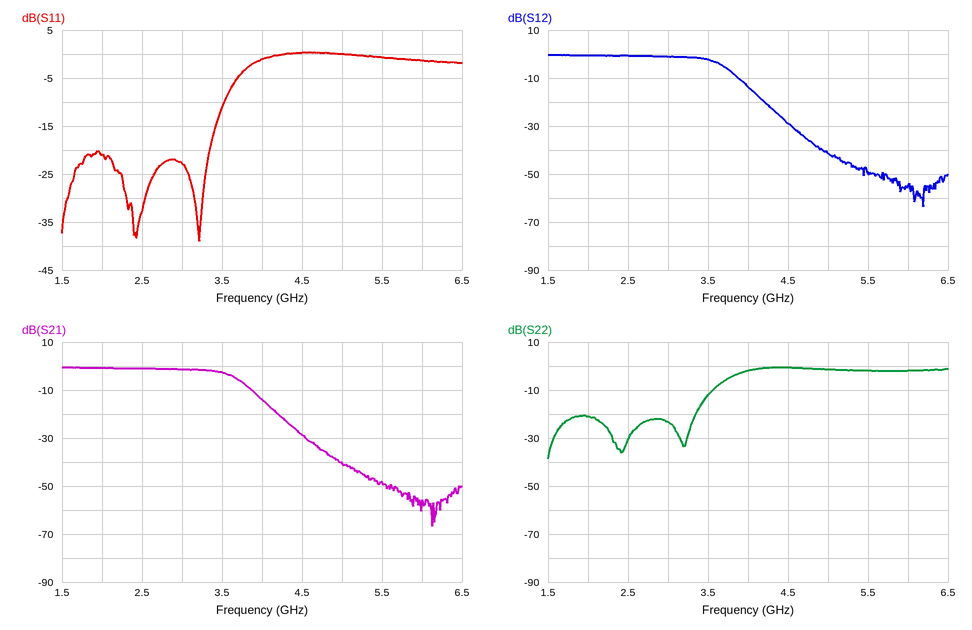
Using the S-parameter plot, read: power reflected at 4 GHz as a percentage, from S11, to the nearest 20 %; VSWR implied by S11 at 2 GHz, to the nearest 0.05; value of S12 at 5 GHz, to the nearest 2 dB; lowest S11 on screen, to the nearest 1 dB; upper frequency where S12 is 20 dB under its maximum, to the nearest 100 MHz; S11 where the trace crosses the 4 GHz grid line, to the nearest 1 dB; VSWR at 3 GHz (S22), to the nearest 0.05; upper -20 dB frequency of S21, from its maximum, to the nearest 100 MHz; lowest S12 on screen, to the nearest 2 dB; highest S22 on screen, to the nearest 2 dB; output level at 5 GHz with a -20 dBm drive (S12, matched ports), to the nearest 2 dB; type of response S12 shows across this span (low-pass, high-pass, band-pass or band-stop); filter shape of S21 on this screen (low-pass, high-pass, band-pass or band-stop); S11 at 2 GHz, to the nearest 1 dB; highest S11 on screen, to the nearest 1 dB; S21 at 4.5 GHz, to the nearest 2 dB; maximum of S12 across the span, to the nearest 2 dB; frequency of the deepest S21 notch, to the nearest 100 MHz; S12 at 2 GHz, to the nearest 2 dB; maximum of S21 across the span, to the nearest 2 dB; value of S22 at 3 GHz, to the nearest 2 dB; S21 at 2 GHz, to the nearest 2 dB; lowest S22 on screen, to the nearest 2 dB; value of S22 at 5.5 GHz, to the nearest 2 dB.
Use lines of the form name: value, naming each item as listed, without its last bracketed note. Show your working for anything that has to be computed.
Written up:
power reflected at 4 GHz as a percentage, from S11, to the nearest 20 %: 10^(-1/10) ≈ 79.4 %, so 80 % to the nearest 20 %
VSWR implied by S11 at 2 GHz, to the nearest 0.05: |Γ| = 10^(-21/20) = 0.0891; VSWR = (1 + 0.0891)/(1 − 0.0891) ≈ 1.20
value of S12 at 5 GHz, to the nearest 2 dB: -42 dB
lowest S11 on screen, to the nearest 1 dB: -39 dB
upper frequency where S12 is 20 dB under its maximum, to the nearest 100 MHz: 4.2 GHz
S11 where the trace crosses the 4 GHz grid line, to the nearest 1 dB: -1 dB
VSWR at 3 GHz (S22), to the nearest 0.05: |Γ| = 10^(-24/20) = 0.0631; VSWR = (1 + 0.0631)/(1 − 0.0631) ≈ 1.13, so 1.15 to the nearest 0.05
upper -20 dB frequency of S21, from its maximum, to the nearest 100 MHz: 4.2 GHz
lowest S12 on screen, to the nearest 2 dB: -64 dB
highest S22 on screen, to the nearest 2 dB: 0 dB
output level at 5 GHz with a -20 dBm drive (S12, matched ports), to the nearest 2 dB: -20 dBm + (-42 dB) = -62 dBm
type of response S12 shows across this span: low-pass
filter shape of S21 on this screen: low-pass
S11 at 2 GHz, to the nearest 1 dB: -21 dB
highest S11 on screen, to the nearest 1 dB: 0 dB
S21 at 4.5 GHz, to the nearest 2 dB: -28 dB
maximum of S12 across the span, to the nearest 2 dB: 0 dB
frequency of the deepest S21 notch, to the nearest 100 MHz: 6.1 GHz
S12 at 2 GHz, to the nearest 2 dB: 0 dB
maximum of S21 across the span, to the nearest 2 dB: 0 dB
value of S22 at 3 GHz, to the nearest 2 dB: -24 dB
S21 at 2 GHz, to the nearest 2 dB: 0 dB
lowest S22 on screen, to the nearest 2 dB: -38 dB
value of S22 at 5.5 GHz, to the nearest 2 dB: -2 dB
